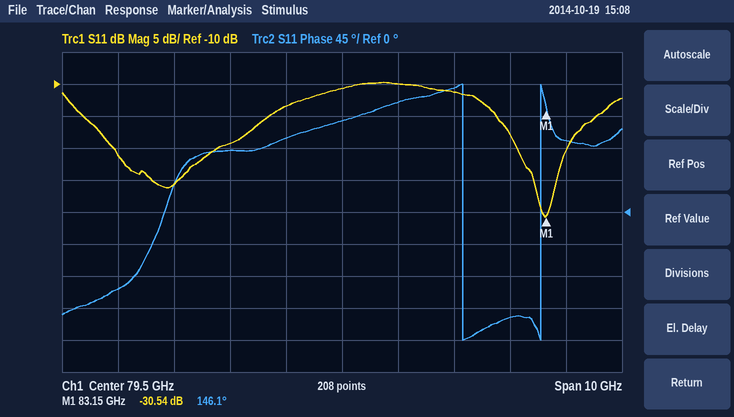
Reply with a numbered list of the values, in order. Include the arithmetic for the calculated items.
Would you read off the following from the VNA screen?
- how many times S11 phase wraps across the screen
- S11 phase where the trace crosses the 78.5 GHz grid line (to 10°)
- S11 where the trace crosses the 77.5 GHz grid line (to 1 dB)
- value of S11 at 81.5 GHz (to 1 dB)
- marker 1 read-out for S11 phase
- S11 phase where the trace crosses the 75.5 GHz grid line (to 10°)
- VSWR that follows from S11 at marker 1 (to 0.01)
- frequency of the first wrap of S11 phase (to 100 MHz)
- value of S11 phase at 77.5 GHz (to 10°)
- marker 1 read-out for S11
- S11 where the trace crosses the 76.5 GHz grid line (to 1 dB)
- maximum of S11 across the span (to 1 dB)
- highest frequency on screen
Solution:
1. 2
2. 100°
3. -19 dB
4. -11 dB
5. 146.1°
6. -110°
7. (1 + 0.0297)/(1 − 0.0297) ≈ 1.06
8. 81.7 GHz
9. 90°
10. -30.54 dB
11. -26 dB
12. -10 dB
13. 84.5 GHz
